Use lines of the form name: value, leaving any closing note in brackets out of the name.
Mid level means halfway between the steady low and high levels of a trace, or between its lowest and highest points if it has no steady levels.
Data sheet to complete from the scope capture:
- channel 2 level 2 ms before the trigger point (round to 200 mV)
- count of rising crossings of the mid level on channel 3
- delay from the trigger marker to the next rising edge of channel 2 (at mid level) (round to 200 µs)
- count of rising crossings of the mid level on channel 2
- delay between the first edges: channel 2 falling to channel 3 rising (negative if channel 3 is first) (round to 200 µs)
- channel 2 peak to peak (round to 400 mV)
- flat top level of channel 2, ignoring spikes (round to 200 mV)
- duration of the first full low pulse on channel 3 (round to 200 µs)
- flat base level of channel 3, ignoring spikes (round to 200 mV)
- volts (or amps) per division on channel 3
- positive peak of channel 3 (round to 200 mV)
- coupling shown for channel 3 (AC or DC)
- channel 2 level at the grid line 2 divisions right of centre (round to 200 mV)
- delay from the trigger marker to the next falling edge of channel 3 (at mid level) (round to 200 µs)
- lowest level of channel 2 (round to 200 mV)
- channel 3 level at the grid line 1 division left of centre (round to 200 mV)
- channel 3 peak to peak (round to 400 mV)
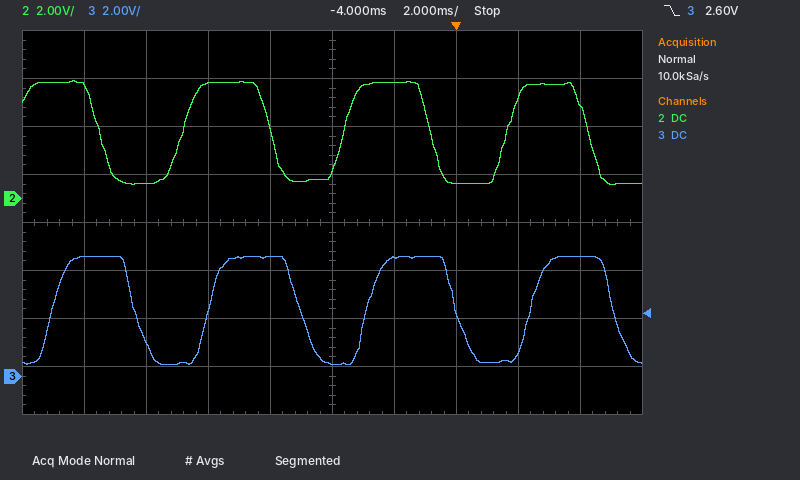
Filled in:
channel 2 level 2 ms before the trigger point: 4.8 V
count of rising crossings of the mid level on channel 3: 4
delay from the trigger marker to the next rising edge of channel 2 (at mid level): 1.6 ms
count of rising crossings of the mid level on channel 2: 3
delay between the first edges: channel 2 falling to channel 3 rising (negative if channel 3 is first): -1.6 ms
channel 2 peak to peak: 4.4 V
flat top level of channel 2, ignoring spikes: 4.8 V
duration of the first full low pulse on channel 3: 2.4 ms
flat base level of channel 3, ignoring spikes: 600 mV
volts (or amps) per division on channel 3: 2 V
positive peak of channel 3: 5.0 V
coupling shown for channel 3: DC
channel 2 level at the grid line 2 divisions right of centre: 600 mV
delay from the trigger marker to the next falling edge of channel 3 (at mid level): 5.0 ms
lowest level of channel 2: 600 mV
channel 3 level at the grid line 1 division left of centre: 5.0 V
channel 3 peak to peak: 4.4 V
